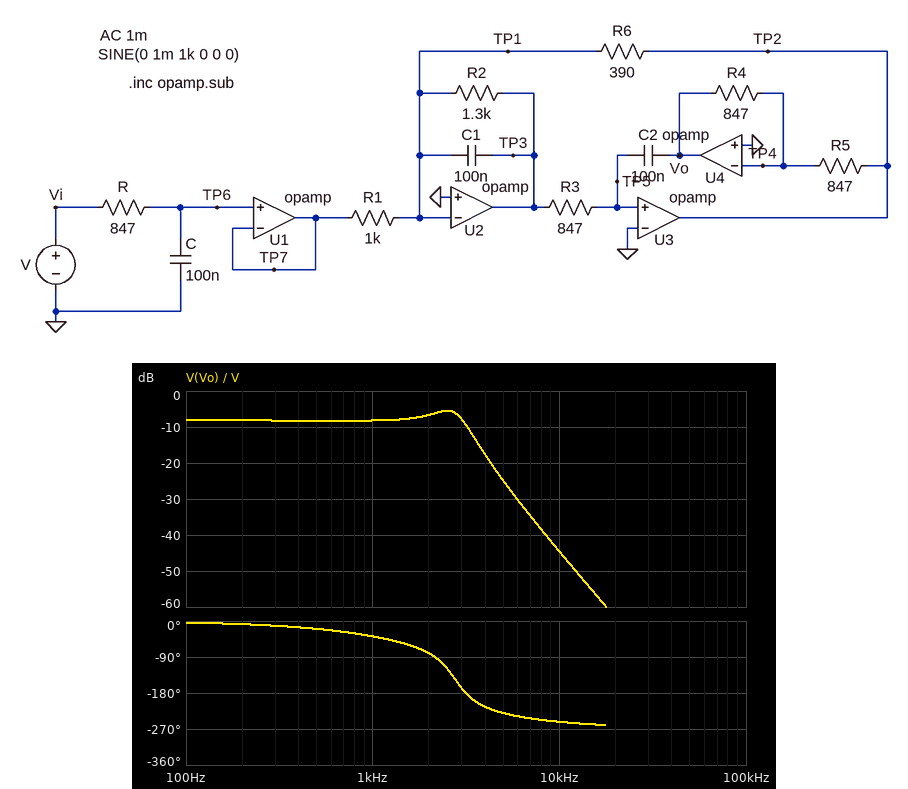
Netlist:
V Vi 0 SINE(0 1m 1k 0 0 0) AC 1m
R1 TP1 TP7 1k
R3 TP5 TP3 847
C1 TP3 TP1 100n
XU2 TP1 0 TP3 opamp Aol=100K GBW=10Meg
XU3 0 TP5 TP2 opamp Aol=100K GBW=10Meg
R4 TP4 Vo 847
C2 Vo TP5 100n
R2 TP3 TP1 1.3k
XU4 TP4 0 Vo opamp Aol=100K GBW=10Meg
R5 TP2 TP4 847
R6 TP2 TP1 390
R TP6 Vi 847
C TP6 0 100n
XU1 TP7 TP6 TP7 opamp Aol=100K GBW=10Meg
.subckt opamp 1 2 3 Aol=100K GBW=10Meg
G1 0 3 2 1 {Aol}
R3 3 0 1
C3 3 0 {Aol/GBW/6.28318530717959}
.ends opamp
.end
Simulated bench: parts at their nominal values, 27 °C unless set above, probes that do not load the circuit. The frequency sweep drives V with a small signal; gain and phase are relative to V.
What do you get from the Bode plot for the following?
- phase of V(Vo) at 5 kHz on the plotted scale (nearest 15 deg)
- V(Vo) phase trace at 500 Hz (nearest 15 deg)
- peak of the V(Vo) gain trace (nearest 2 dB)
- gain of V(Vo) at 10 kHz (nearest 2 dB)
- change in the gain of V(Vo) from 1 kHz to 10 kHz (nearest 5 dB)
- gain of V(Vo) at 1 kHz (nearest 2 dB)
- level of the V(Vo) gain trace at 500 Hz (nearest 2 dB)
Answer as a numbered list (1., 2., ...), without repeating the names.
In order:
1. -225 deg
2. -15 deg
3. -6 dB
4. -44 dB
5. -35 dB
6. -8 dB
7. -8 dB
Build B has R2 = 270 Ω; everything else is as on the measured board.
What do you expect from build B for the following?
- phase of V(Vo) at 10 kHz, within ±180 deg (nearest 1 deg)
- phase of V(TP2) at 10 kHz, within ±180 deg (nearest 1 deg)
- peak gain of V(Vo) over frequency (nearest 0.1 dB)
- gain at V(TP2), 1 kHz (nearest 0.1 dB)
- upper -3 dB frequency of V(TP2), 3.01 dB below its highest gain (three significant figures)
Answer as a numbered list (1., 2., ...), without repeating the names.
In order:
1. 133 deg
2. -47 deg
3. -8.2 dB
4. -10.6 dB
5. 1.14 kHz
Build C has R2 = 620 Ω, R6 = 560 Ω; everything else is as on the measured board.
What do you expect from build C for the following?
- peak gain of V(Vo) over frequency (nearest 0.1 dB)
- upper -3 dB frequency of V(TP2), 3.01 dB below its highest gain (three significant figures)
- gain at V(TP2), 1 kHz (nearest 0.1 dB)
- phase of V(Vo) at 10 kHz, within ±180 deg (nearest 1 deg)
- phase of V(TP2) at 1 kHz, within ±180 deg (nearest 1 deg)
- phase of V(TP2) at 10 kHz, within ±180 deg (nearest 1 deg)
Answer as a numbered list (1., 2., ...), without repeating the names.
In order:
1. -5.0 dB
2. 1.95 kHz
3. -5.6 dB
4. 116 deg
5. 121 deg
6. -64 deg
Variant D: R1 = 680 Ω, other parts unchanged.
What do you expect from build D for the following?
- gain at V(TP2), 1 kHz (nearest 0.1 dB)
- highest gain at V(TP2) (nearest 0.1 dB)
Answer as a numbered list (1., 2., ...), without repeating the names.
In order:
1. -4.8 dB
2. -2.1 dB
